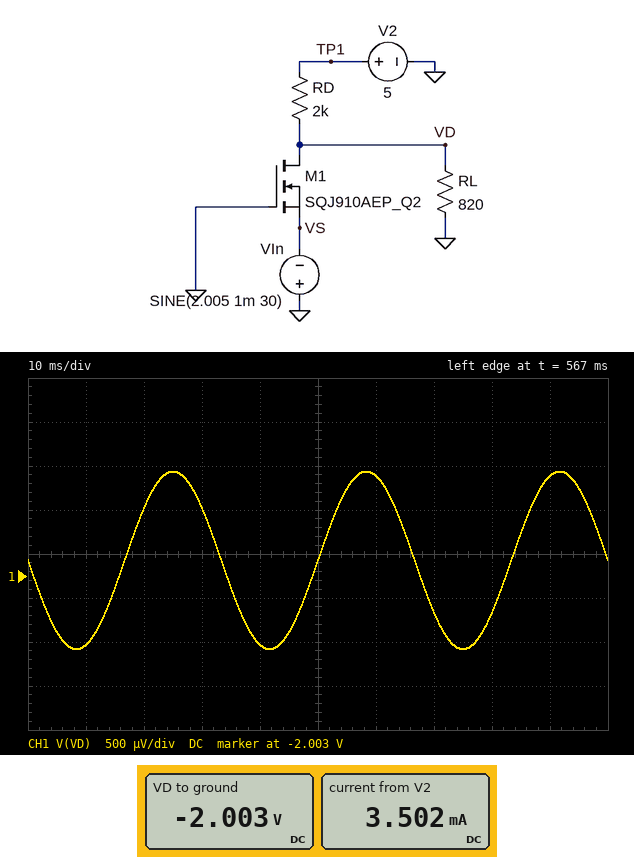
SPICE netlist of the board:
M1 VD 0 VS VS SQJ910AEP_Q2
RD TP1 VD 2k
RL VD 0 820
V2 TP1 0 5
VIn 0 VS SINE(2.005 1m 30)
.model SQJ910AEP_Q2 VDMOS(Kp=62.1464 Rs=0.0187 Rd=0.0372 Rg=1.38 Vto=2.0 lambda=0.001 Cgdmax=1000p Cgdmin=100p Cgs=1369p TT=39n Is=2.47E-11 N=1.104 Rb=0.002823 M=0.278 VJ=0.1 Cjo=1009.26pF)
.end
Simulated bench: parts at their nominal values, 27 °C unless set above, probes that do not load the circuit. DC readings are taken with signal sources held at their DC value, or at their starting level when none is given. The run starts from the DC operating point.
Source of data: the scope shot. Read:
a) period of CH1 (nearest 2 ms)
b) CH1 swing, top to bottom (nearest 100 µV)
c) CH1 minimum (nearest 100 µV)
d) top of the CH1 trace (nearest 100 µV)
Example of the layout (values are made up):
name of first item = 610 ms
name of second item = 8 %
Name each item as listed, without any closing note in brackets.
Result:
period of CH1 = 34 ms
CH1 swing, top to bottom = 2.0 mV
CH1 minimum = -2.0043 V
top of the CH1 trace = -2.0023 V
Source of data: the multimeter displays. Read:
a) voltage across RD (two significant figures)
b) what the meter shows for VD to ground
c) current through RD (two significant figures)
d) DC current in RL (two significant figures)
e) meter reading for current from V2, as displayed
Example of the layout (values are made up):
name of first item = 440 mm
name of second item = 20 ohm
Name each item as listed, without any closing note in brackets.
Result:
voltage across RD = 7.0 V
what the meter shows for VD to ground = -2.003 V
current through RD = 3.5 mA
DC current in RL = 2.4 mA
meter reading for current from V2, as displayed = 3.502 mA
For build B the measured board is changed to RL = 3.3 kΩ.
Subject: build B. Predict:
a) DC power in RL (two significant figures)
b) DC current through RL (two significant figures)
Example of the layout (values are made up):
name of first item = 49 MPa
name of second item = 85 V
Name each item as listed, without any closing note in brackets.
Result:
DC power in RL = 1.2 mW
DC current through RL = 610 µA
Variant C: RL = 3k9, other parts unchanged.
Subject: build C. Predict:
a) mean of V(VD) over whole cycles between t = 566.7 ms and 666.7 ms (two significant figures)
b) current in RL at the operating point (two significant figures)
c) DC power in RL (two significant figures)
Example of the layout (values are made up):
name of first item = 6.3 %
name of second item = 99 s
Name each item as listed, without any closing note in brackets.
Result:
mean of V(VD) over whole cycles between t = 566.7 ms and 666.7 ms = -2.0 V
current in RL at the operating point = 510 µA
DC power in RL = 1.0 mW
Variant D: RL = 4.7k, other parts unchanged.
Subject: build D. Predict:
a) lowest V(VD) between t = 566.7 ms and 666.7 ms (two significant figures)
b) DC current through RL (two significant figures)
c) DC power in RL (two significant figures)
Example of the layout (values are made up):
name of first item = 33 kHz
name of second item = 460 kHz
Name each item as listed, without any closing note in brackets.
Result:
lowest V(VD) between t = 566.7 ms and 666.7 ms = -2.0 V
DC current through RL = 430 µA
DC power in RL = 850 µW
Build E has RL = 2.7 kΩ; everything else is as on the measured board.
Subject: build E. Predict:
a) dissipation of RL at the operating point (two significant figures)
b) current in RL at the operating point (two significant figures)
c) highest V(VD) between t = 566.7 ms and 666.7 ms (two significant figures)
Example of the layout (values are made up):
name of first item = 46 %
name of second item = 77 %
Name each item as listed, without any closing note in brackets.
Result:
dissipation of RL at the operating point = 1.5 mW
current in RL at the operating point = 740 µA
highest V(VD) between t = 566.7 ms and 666.7 ms = -2.0 V
